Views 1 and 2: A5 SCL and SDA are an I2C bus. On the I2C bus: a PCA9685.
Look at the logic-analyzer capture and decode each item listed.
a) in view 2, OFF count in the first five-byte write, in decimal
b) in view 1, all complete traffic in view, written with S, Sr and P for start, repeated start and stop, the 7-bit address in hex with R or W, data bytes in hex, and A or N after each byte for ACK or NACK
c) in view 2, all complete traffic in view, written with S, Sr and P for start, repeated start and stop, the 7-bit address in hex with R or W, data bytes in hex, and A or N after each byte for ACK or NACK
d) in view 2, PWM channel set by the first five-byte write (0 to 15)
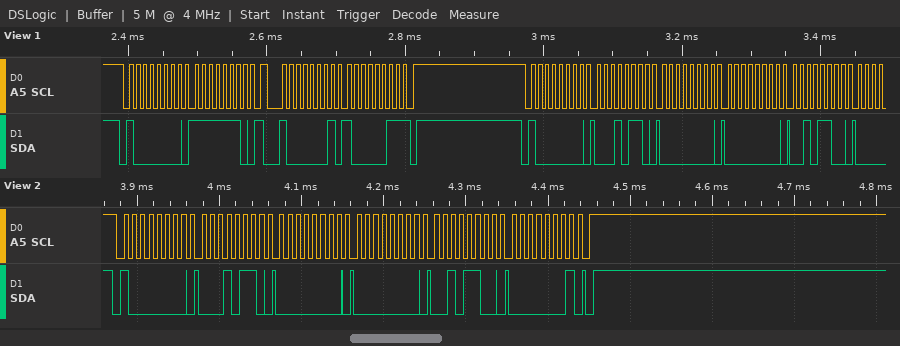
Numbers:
300
S 40W A FE A Sr 40R A 83 N P S 40W A 16 A 00 A 00 A 2C A
S 40W A 16 A 00 A 00 A 2C A 01 A P
4
